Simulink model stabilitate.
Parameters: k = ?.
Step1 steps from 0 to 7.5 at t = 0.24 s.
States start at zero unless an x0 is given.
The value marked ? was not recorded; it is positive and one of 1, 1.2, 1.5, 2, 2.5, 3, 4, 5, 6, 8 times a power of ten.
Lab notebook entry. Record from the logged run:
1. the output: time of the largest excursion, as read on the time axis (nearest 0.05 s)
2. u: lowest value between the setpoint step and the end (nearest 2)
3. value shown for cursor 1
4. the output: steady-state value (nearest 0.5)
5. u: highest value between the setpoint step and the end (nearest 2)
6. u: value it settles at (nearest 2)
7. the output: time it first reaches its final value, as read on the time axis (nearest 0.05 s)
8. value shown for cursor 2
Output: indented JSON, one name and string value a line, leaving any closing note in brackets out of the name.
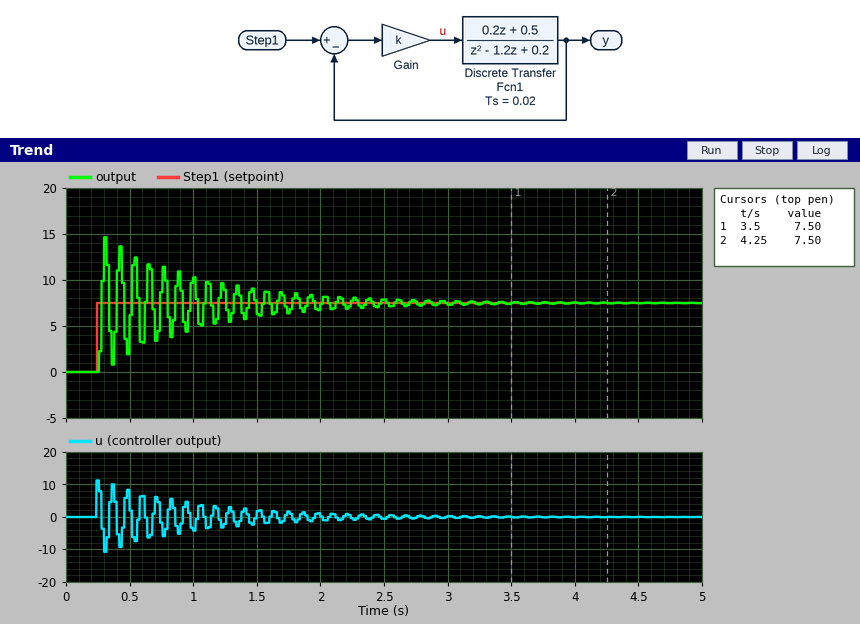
{
  "the output: time of the largest excursion, as read on the time axis": "0.30 s",
  "u: lowest value between the setpoint step and the end": "-10",
  "value shown for cursor 1": "7.50",
  "the output: steady-state value": "7.5",
  "u: highest value between the setpoint step and the end": "12",
  "u: value it settles at": "0",
  "the output: time it first reaches its final value, as read on the time axis": "0.30 s",
  "value shown for cursor 2": "7.50"
}
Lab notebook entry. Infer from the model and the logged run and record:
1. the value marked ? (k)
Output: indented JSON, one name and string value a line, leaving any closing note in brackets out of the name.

{
  "the value marked ?": "1.5"
}
